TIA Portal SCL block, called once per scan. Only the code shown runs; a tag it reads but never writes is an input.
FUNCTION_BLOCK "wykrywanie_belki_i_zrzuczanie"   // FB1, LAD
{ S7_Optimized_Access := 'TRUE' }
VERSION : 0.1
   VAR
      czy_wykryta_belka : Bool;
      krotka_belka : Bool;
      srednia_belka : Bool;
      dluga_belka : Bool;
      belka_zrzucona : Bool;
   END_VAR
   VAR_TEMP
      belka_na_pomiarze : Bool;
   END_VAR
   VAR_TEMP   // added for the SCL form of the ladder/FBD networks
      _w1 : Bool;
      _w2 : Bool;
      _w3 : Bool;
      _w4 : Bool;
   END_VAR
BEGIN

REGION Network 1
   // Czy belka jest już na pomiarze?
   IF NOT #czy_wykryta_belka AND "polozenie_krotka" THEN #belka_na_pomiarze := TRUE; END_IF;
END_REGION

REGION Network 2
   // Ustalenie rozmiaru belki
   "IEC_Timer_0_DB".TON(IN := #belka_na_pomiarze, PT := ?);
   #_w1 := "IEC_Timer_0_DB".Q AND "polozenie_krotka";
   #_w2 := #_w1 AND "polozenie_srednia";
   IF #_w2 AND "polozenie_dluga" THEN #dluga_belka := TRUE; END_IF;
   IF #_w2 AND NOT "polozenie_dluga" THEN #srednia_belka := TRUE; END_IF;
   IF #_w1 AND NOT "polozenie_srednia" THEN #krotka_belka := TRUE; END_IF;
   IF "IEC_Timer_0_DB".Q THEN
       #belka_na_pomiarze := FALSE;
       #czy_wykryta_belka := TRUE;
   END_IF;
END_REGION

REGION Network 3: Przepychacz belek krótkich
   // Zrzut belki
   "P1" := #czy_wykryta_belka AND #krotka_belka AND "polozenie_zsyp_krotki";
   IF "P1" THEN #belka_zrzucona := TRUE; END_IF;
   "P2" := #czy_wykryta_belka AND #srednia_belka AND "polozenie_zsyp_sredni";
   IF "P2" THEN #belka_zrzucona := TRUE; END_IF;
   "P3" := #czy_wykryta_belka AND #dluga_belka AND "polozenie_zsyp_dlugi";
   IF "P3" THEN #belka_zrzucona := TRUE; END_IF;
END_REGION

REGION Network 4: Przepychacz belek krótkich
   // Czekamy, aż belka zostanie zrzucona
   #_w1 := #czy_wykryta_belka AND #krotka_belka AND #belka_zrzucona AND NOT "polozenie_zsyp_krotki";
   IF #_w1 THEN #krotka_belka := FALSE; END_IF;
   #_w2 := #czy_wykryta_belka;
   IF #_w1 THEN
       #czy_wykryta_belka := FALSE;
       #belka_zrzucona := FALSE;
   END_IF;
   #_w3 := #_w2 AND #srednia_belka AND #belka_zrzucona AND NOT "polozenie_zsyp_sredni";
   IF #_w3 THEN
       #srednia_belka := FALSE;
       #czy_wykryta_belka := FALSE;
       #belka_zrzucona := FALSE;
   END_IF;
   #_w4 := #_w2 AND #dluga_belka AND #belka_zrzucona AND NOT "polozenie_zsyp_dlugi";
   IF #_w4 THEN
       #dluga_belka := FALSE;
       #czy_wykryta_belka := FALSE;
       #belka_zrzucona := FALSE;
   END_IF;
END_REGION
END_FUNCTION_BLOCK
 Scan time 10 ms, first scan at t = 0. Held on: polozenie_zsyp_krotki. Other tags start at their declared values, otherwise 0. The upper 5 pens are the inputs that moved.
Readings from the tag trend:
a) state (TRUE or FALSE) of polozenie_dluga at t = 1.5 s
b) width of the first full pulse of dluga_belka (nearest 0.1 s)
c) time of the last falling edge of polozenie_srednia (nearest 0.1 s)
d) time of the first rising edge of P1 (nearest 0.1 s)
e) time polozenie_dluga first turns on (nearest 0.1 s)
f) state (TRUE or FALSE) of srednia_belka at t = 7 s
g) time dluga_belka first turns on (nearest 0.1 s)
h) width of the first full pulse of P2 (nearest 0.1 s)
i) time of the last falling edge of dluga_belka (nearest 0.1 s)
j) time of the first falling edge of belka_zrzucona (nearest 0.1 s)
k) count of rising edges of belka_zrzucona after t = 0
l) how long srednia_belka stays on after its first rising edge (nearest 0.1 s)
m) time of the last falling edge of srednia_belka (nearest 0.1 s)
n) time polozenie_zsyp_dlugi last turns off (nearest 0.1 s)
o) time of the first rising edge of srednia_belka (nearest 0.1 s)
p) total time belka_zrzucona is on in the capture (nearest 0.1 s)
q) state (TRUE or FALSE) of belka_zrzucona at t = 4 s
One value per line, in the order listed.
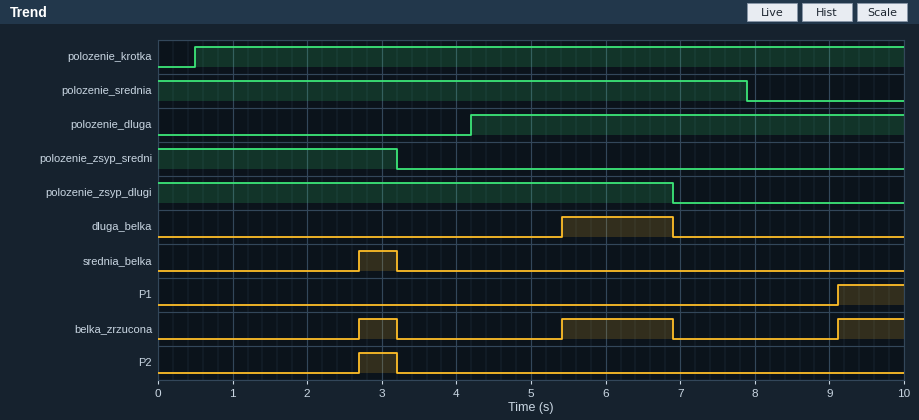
FALSE
1.5 s
7.9 s
9.1 s
4.2 s
FALSE
5.4 s
0.5 s
6.9 s
3.2 s
3
0.5 s
3.2 s
6.9 s
2.7 s
2.9 s
FALSE
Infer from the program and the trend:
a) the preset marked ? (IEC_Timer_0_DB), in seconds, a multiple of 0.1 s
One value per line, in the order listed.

2.2 s
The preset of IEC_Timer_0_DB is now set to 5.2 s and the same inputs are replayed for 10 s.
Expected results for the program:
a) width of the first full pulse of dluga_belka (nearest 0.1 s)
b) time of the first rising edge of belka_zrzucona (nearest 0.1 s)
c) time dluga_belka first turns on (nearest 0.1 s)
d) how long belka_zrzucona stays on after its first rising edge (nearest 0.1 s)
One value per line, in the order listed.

1.2 s
5.7 s
5.7 s
1.2 s
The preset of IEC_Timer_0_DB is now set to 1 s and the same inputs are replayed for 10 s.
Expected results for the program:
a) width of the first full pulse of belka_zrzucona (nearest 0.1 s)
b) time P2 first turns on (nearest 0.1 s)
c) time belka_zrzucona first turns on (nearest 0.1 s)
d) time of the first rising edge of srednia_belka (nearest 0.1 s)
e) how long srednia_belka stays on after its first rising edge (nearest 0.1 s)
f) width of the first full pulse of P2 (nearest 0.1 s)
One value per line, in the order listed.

1.7 s
1.5 s
1.5 s
1.5 s
1.7 s
1.7 s
